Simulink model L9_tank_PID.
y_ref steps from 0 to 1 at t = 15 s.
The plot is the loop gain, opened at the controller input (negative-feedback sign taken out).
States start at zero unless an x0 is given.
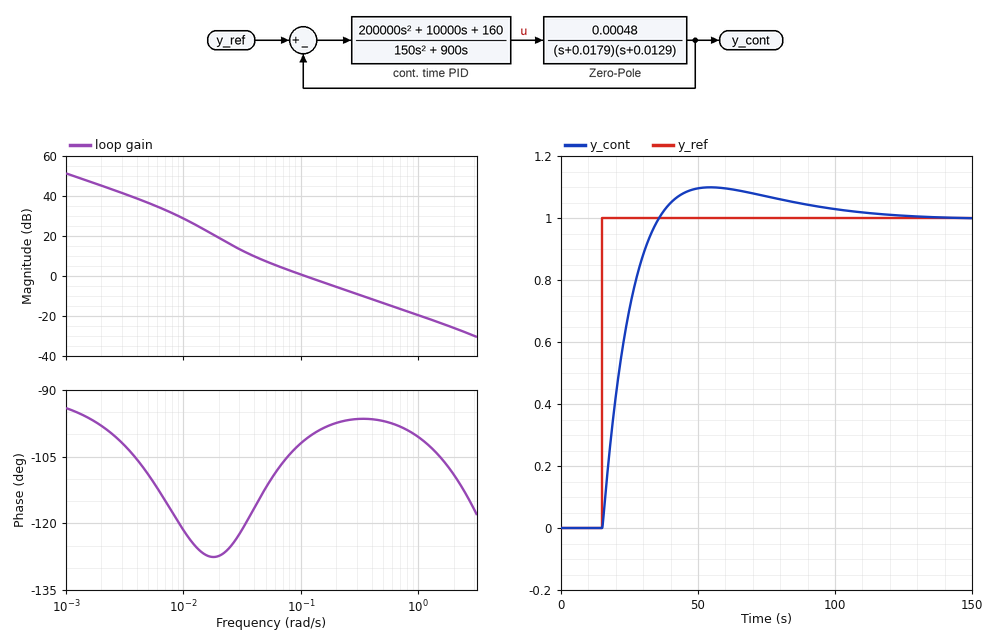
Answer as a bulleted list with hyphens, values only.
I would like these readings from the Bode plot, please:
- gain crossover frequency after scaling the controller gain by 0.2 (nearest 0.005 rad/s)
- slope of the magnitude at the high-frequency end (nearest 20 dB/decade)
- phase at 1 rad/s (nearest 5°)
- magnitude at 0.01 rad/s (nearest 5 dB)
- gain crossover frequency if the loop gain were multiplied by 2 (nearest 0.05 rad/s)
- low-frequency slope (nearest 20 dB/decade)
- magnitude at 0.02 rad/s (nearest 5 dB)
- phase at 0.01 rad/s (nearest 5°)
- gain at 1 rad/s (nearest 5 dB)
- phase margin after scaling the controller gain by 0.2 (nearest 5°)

- 0.030 rad/s
- -20 dB/decade
- -100°
- 30 dB
- 0.20 rad/s
- -20 dB/decade
- 20 dB
- -120°
- -20 dB
- 55°
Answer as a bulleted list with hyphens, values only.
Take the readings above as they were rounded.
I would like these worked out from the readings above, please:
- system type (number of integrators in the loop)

- 1
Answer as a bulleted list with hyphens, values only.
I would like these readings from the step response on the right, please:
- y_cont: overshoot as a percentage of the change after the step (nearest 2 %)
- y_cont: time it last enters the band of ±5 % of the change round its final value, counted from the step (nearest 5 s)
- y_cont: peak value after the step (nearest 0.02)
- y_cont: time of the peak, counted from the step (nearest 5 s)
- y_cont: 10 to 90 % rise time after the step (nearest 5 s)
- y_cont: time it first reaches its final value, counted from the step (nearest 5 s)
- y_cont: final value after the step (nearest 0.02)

- 10 %
- 70 s
- 1.10
- 40 s
- 15 s
- 20 s
- 1.00
